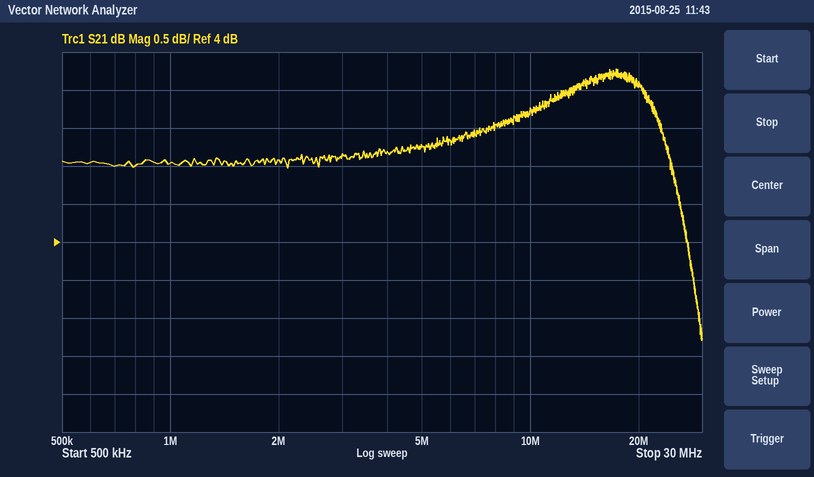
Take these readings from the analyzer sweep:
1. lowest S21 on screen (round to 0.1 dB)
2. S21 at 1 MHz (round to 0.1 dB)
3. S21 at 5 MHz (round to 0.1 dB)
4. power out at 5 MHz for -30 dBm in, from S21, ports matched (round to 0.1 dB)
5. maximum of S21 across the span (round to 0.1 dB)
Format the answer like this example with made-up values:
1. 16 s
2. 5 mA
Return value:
1. 2.7 dB
2. 5.0 dB
3. 5.3 dB
4. -24.7 dBm
5. 6.3 dB
